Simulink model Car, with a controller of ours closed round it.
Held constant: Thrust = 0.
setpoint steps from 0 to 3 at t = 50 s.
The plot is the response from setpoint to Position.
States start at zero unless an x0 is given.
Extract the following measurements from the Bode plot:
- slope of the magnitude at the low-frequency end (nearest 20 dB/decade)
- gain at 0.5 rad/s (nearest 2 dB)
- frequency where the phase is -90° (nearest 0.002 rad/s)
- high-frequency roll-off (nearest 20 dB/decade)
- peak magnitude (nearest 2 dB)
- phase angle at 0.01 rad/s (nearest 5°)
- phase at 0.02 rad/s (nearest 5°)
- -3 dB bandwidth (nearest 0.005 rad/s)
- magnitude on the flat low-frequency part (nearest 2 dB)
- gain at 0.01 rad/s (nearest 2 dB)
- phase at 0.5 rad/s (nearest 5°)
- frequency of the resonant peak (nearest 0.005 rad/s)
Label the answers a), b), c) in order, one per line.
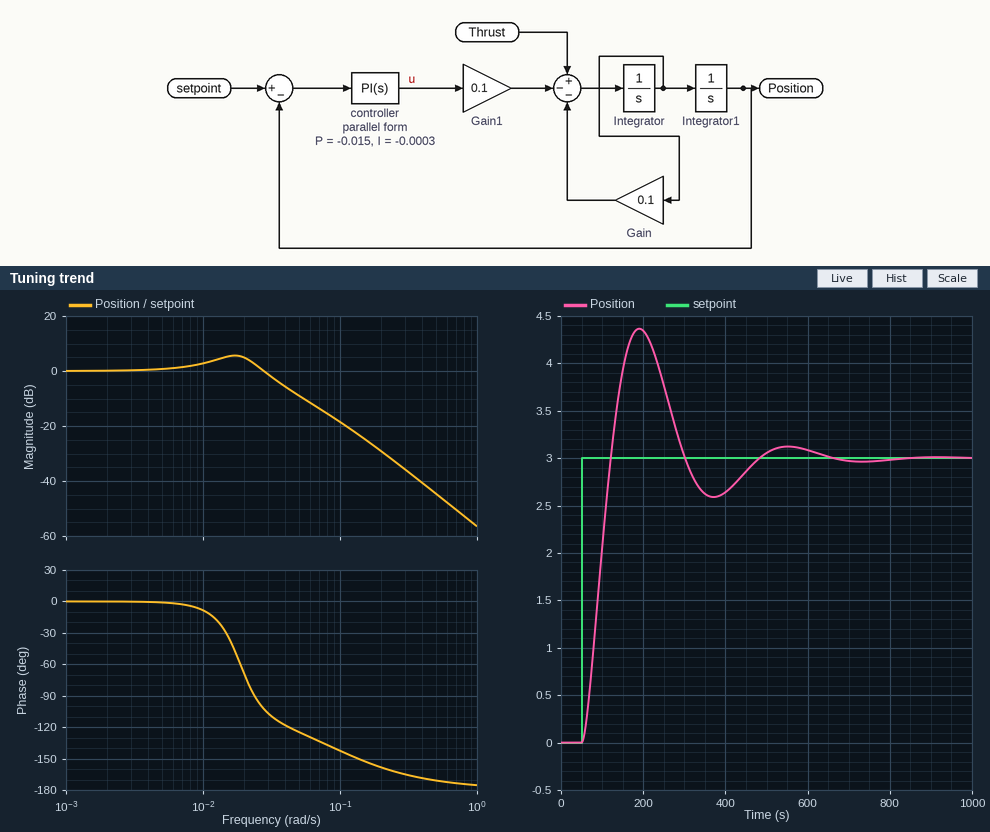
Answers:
a) 0 dB/decade
b) -44 dB
c) 0.024 rad/s
d) -40 dB/decade
e) 6 dB
f) -10°
g) -70°
h) 0.035 rad/s
i) 0 dB
j) 2 dB
k) -170°
l) 0.015 rad/s
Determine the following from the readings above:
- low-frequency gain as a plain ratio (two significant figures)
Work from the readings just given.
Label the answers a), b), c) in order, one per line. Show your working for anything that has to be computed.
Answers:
a) 10^(0 / 20) = 1.0
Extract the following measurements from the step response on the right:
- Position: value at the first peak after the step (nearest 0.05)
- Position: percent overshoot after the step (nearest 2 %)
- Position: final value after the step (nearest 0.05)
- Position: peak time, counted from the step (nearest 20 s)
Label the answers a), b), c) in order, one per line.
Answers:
a) 4.35
b) 46 %
c) 3.00
d) 140 s
